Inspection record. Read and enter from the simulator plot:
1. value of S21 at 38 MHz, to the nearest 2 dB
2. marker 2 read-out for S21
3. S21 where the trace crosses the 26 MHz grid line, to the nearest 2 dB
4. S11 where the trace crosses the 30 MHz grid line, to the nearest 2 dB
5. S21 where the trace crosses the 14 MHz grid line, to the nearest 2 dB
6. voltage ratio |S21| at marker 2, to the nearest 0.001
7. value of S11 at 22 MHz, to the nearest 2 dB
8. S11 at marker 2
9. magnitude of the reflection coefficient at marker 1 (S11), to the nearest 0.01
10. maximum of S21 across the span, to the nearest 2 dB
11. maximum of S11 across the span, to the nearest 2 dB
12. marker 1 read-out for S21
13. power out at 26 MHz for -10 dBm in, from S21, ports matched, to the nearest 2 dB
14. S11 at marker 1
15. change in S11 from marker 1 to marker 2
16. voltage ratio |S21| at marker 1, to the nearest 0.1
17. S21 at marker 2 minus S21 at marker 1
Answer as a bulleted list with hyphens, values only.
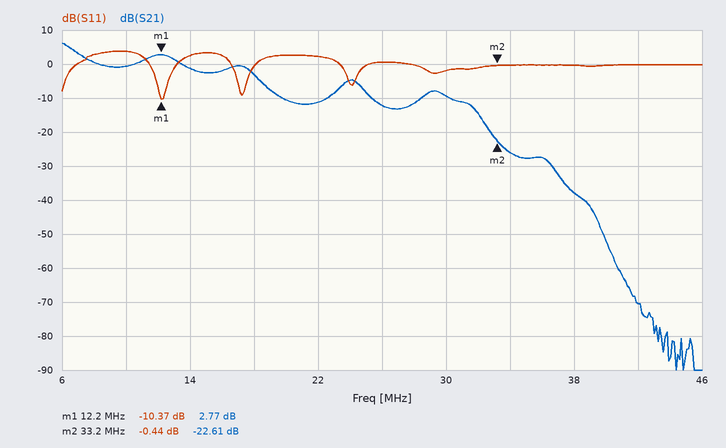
- -38 dB
- -22.61 dB
- -12 dB
- -2 dB
- -2 dB
- 0.074
- 2 dB
- -0.44 dB
- 0.30
- 6 dB
- 4 dB
- 2.77 dB
- -22 dBm
- -10.37 dB
- 9.93 dB
- 1.4
- -25.38 dB
